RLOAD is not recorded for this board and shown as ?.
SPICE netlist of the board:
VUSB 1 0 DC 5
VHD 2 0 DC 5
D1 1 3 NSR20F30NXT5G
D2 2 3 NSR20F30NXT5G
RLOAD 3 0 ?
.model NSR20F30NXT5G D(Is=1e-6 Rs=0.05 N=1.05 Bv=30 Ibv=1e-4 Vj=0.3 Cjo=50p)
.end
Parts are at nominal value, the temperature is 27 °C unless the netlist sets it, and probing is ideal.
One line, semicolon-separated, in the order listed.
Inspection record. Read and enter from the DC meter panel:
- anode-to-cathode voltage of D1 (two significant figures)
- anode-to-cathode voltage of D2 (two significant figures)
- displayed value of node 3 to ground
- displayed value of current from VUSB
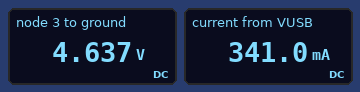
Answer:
360 mV; 360 mV; 4.637 V; 341.0 mA
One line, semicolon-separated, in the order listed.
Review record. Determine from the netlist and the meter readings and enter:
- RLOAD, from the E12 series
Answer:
6.8 Ω
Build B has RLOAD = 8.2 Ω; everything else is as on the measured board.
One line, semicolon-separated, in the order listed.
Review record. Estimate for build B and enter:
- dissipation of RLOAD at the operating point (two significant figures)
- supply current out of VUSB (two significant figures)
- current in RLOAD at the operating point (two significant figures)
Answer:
2.6 W; 280 mA; 570 mA
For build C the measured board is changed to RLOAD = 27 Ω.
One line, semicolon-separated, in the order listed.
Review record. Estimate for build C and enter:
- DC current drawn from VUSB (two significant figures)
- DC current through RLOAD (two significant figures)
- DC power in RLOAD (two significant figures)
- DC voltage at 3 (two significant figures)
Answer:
87 mA; 170 mA; 810 mW; 4.7 V
